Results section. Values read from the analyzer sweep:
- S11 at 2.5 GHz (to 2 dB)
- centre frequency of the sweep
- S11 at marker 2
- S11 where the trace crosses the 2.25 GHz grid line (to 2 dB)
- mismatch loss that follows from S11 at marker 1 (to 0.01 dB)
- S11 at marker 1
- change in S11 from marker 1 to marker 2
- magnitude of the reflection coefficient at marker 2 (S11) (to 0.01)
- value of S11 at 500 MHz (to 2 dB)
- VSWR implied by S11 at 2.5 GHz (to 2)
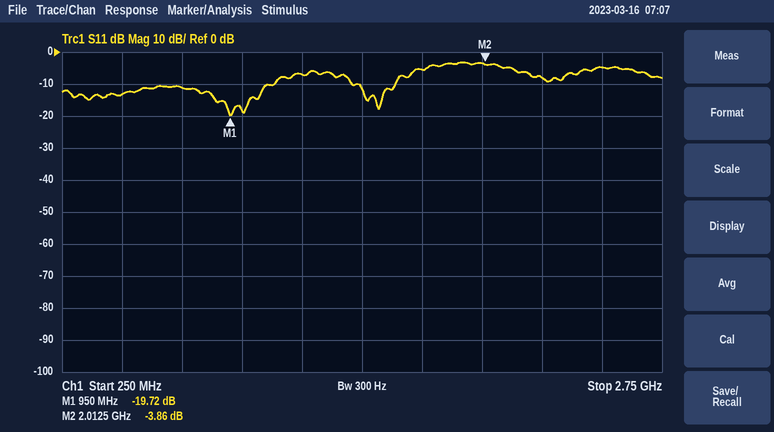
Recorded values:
-4 dB
1.5 GHz
-3.86 dB
-8 dB
0.05 dB
-19.72 dB
15.86 dB
0.64
-14 dB
4
